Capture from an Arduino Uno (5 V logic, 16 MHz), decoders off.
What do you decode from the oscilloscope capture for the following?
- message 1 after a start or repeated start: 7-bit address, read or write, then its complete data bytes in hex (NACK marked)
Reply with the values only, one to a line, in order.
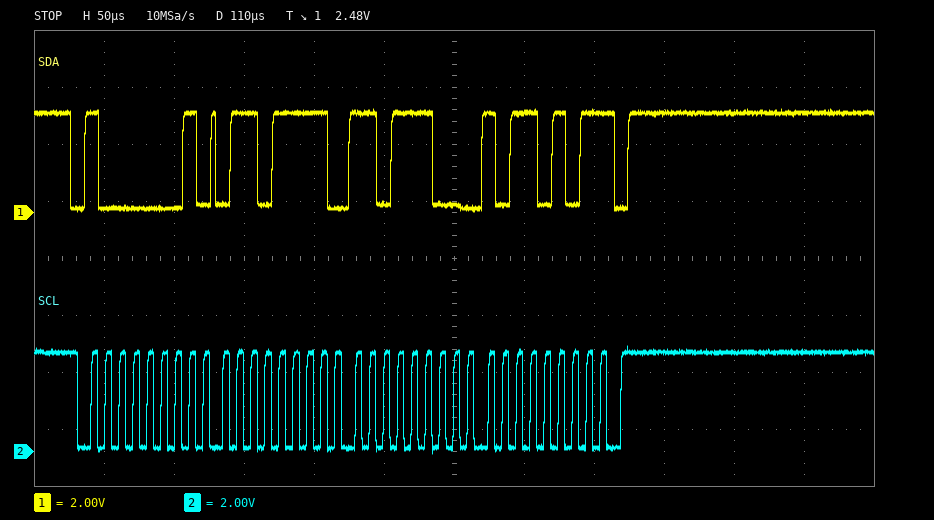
0x40 read: 6F DC B5 NACK
